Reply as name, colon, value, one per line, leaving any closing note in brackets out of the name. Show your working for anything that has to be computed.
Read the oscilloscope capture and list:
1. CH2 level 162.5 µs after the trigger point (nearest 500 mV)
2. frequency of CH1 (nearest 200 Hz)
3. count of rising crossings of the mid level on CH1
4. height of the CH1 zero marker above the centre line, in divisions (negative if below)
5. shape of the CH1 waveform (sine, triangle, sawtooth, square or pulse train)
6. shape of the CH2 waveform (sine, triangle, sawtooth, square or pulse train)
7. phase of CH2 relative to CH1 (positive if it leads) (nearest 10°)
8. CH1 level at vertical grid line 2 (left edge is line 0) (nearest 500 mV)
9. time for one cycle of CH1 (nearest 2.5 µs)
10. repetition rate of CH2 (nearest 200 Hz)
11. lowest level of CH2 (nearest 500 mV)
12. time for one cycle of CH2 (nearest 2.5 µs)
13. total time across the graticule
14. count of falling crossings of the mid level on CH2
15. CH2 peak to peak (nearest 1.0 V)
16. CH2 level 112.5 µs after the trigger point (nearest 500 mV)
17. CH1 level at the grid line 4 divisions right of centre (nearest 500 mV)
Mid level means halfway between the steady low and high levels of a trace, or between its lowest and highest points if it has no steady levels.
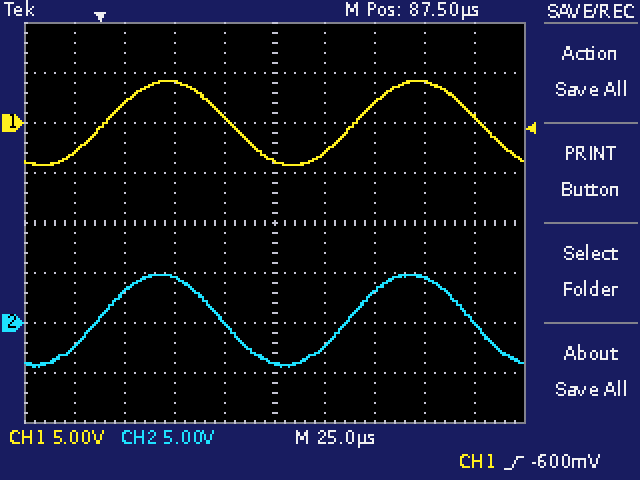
CH2 level 162.5 µs after the trigger point: 4.5 V
frequency of CH1: 1 / 125.0 µs ≈ 8.0 kHz
count of rising crossings of the mid level on CH1: 2
height of the CH1 zero marker above the centre line, in divisions: +2.0 div
shape of the CH1 waveform: sine
shape of the CH2 waveform: sine
phase of CH2 relative to CH1 (positive if it leads): +10°
CH1 level at vertical grid line 2 (left edge is line 0): 2.0 V
time for one cycle of CH1: 125.0 µs
repetition rate of CH2: 1 / 125.0 µs ≈ 8.0 kHz
lowest level of CH2: -4.5 V
time for one cycle of CH2: 125.0 µs
total time across the graticule: 250 µs
count of falling crossings of the mid level on CH2: 2
CH2 peak to peak: 9.0 V
CH2 level 112.5 µs after the trigger point: -2.5 V
CH1 level at the grid line 4 divisions right of centre: 500 mV
